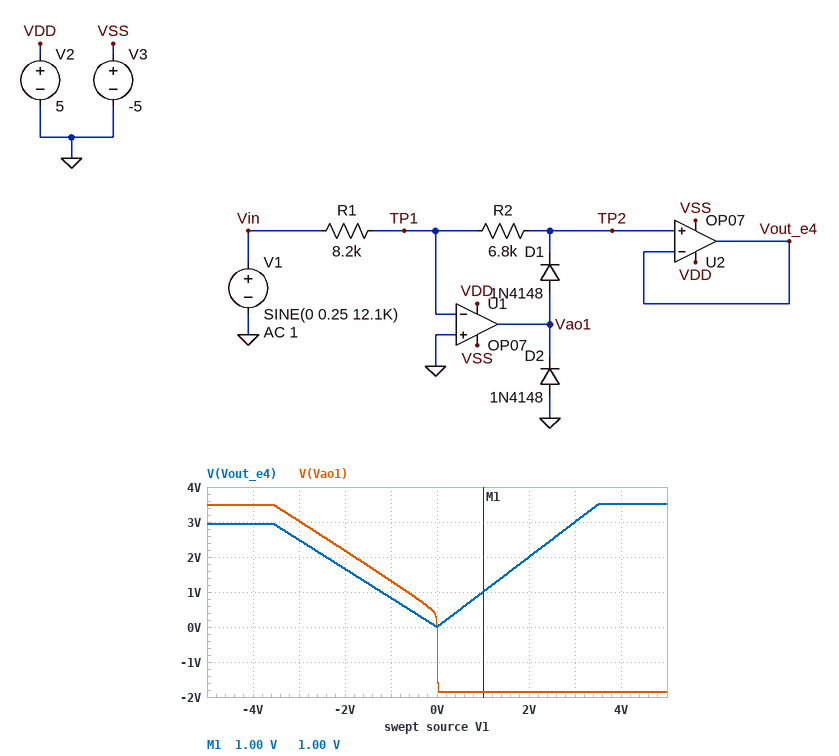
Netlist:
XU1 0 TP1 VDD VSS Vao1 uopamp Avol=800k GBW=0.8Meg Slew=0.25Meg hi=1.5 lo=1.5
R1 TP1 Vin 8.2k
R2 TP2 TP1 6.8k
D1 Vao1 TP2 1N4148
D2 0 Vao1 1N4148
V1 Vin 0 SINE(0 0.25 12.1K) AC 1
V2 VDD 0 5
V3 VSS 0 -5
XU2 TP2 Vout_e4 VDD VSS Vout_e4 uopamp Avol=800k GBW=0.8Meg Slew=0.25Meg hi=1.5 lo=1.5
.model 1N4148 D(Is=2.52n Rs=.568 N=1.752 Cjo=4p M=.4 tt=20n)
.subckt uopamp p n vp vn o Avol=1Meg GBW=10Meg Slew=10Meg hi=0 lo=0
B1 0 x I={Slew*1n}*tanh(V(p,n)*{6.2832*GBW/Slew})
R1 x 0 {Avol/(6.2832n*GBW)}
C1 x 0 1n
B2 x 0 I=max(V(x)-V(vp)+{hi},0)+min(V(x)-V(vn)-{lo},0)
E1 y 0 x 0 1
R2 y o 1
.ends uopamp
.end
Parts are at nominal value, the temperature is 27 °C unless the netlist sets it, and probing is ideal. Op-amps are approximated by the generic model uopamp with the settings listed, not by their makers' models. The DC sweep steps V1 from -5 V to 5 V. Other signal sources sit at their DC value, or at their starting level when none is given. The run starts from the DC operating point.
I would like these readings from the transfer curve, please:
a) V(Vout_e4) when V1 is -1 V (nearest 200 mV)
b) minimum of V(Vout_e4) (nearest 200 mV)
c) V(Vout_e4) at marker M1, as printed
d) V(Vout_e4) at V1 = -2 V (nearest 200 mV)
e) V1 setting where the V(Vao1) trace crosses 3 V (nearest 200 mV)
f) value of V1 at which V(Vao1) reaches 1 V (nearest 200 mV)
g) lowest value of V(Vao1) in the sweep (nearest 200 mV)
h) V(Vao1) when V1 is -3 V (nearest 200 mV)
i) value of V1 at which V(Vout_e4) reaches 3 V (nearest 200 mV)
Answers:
800 mV
0 V
1.00 V
1.6 V
-3.0 V
-600 mV
-1.8 V
3.0 V
3.0 V
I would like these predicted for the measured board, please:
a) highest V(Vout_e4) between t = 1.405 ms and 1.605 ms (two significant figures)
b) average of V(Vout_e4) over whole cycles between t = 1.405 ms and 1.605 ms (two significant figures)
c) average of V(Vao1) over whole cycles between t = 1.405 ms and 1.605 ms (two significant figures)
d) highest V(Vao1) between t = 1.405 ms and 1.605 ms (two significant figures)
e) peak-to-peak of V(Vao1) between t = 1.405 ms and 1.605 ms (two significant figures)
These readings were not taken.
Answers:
250 mV
92 mV
-800 mV
630 mV
2.5 V
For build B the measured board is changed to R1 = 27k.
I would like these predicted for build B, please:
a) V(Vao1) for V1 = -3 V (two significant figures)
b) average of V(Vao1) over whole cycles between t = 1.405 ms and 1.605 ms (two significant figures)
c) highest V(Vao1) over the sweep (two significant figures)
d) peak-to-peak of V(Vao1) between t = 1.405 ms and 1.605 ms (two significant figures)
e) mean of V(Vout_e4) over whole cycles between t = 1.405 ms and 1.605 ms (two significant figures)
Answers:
1.2 V
-840 mV
1.8 V
2.3 V
64 mV
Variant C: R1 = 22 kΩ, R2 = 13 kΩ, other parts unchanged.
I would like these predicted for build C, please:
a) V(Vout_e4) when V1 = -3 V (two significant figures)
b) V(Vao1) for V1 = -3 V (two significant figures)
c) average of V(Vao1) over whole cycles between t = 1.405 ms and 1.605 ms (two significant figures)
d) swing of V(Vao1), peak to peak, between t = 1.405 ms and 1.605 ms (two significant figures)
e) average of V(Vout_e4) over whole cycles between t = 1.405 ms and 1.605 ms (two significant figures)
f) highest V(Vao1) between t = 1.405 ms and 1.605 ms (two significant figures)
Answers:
1.8 V
2.3 V
-820 mV
2.4 V
81 mV
530 mV
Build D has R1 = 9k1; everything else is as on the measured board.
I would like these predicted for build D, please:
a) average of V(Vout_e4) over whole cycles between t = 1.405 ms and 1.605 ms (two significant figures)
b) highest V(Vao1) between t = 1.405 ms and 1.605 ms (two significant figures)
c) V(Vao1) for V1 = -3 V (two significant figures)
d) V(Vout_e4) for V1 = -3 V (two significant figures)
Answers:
88 mV
610 mV
2.8 V
2.2 V
